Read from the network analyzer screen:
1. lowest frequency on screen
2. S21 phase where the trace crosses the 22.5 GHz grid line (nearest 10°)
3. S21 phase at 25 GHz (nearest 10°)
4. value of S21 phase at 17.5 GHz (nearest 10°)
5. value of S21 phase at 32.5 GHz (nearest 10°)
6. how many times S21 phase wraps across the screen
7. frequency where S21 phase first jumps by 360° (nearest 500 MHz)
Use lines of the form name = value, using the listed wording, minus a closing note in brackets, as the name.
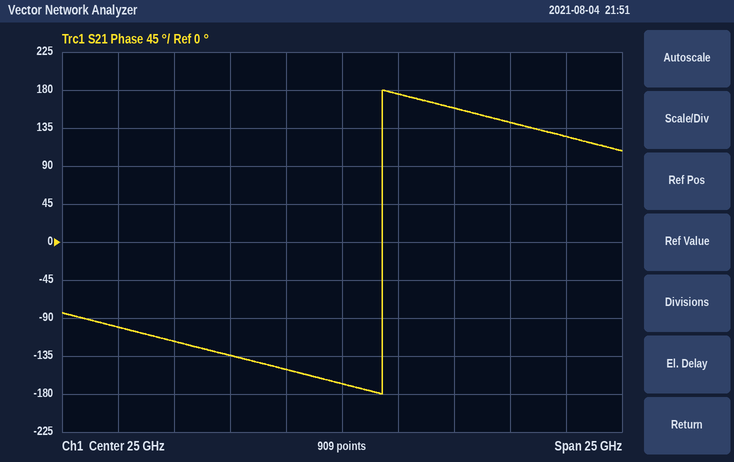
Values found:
lowest frequency on screen = 12.5 GHz
S21 phase where the trace crosses the 22.5 GHz grid line = -150°
S21 phase at 25 GHz = -170°
value of S21 phase at 17.5 GHz = -120°
value of S21 phase at 32.5 GHz = 140°
how many times S21 phase wraps across the screen = 1
frequency where S21 phase first jumps by 360° = 27.0 GHz
